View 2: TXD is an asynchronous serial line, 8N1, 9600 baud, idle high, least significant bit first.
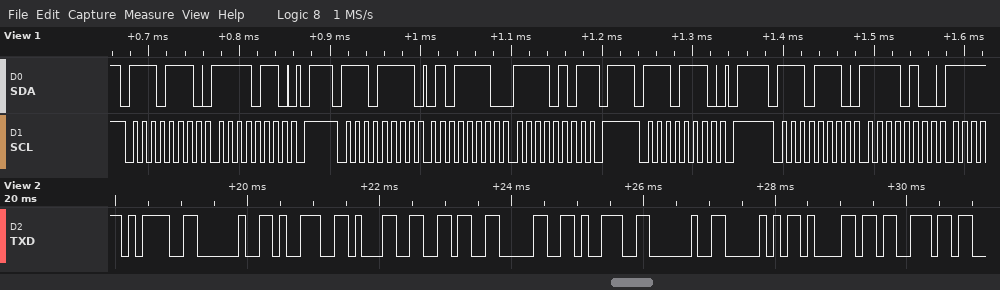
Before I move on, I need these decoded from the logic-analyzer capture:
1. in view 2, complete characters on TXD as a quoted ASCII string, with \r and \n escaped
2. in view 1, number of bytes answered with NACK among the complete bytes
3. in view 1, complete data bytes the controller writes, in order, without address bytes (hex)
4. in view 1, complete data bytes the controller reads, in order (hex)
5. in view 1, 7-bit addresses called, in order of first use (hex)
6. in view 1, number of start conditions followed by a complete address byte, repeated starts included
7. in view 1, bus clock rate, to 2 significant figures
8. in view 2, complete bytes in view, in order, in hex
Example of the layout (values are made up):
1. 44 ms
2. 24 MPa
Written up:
1. "= 91609 Pas"
2. 1
3. F6 F4
4. 5E F5
5. 0x77
6. 4
7. 100 kHz
8. 3D 20 39 31 36 30 39 20 50 61 73
